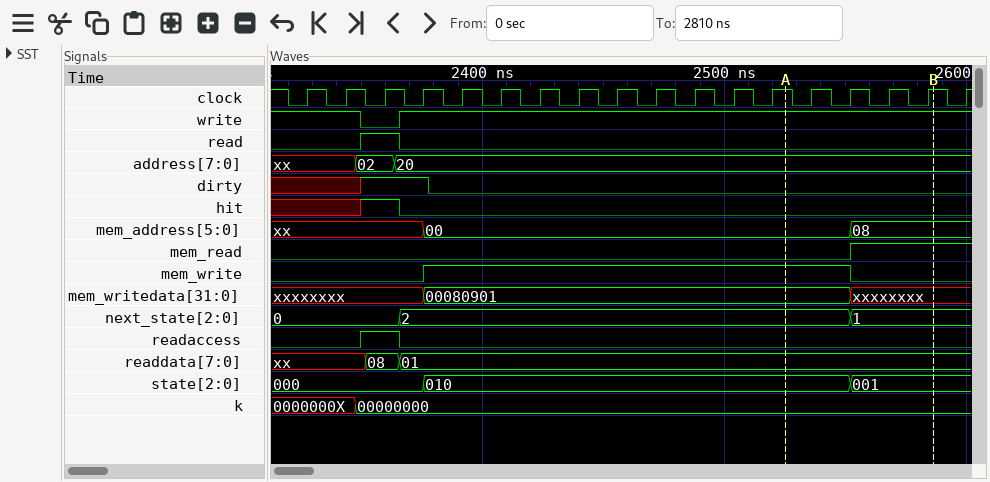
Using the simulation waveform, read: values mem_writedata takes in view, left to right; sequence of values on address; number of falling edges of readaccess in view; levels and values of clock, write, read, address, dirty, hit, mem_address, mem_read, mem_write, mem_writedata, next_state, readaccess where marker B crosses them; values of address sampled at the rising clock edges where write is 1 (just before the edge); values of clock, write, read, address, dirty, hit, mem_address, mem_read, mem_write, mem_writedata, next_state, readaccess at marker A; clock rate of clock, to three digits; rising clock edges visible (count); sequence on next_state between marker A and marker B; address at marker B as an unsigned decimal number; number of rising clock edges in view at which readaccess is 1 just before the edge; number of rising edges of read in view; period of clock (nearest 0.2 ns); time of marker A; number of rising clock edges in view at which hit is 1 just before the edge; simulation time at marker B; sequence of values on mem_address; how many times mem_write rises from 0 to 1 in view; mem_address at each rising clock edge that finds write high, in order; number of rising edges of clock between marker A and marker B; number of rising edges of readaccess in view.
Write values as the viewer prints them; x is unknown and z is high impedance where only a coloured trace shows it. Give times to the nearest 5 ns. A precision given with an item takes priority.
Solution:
xxxxxxxx, 00080901, xxxxxxxx
xx, 02, 20
1
clock=1, write=1, read=0, address=20, dirty=0, hit=0, mem_address=08, mem_read=1, mem_write=0, mem_writedata=xxxxxxxx, next_state=1, readaccess=0
xx, xx, 20, 20, 20, 20, 20, 20, 20, 20, 20, 20, 20, 20, 20, 20, 20
clock=1, write=1, read=0, address=20, dirty=0, hit=0, mem_address=00, mem_read=0, mem_write=1, mem_writedata=00080901, next_state=2, readaccess=0
62.5 MHz
18
2, 1
32
1
1
16 ns
2525 ns
1
2585 ns
xx, 00, 08
1
xx, xx, xx, 00, 00, 00, 00, 00, 00, 00, 00, 00, 00, 00, 08, 08, 08
4
1
